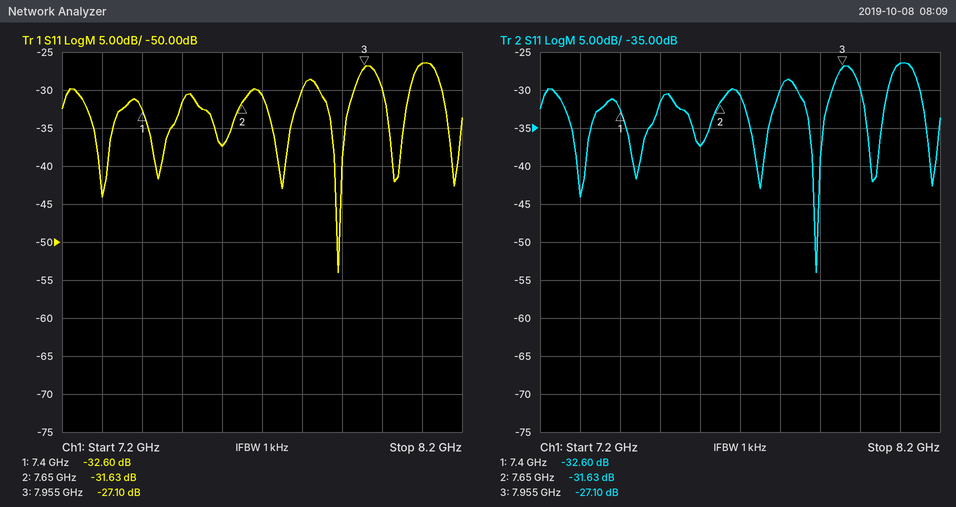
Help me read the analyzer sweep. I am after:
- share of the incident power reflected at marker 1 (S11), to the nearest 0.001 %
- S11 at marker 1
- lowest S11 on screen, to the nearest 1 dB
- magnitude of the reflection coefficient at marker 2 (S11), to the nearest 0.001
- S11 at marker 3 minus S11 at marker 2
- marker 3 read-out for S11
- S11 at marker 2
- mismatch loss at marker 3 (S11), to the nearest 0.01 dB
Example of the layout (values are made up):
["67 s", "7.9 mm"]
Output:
["0.055 %", "-32.60 dB", "-54 dB", "0.026", "4.53 dB", "-27.10 dB", "-31.63 dB", "0.01 dB"]
